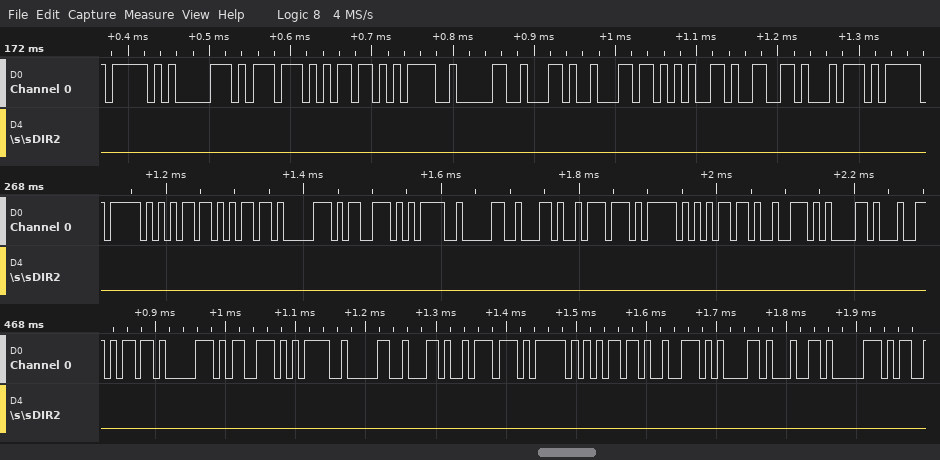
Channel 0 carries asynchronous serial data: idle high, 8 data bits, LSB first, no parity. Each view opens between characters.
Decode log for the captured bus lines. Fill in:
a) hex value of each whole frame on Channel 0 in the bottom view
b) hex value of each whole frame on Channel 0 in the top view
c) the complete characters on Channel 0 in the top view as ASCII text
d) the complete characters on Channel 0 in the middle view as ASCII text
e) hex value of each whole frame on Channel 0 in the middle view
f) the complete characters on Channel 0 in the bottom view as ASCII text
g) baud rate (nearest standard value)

6D, 70, 73, 3D, 30, 2C, 77, 5F, 6D, 72, 61, 64, 70
5F, 70, 77, 6D, 3D, 30, 2C, 6C, 65, 66, 74
"_pwm=0,left"
"_mmps=0,w_mra"
5F, 6D, 6D, 70, 73, 3D, 30, 2C, 77, 5F, 6D, 72, 61
"mps=0,w_mradp"
115200 baud
